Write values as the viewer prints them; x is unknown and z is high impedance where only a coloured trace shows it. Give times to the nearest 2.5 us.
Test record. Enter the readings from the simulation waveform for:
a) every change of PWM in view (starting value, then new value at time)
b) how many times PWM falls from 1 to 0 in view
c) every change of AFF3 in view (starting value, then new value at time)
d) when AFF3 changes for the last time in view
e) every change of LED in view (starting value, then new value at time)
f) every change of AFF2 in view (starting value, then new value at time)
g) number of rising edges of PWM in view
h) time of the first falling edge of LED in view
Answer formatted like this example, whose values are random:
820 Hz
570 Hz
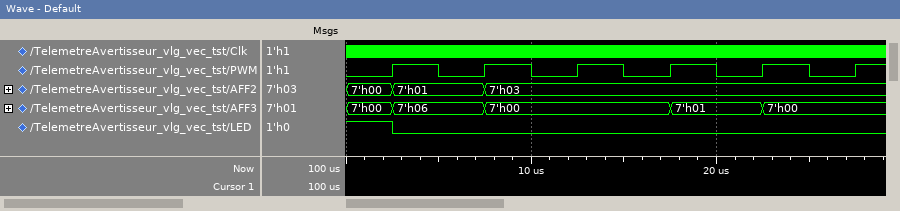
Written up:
0, 1 at 2.5 us, 0 at 5 us, 1 at 7.5 us, 0 at 10 us, 1 at 12.5 us, 0 at 15 us, 1 at 17.5 us, 0 at 20 us, 1 at 22.5 us, 0 at 25 us, 1 at 27.5 us
5
7'h00, 7'h06 at 2.5 us, 7'h00 at 7.5 us, 7'h01 at 17.5 us, 7'h00 at 22.5 us
22.5 us
1, 0 at 2.5 us
7'h00, 7'h01 at 2.5 us, 7'h03 at 7.5 us
6
2.5 us
